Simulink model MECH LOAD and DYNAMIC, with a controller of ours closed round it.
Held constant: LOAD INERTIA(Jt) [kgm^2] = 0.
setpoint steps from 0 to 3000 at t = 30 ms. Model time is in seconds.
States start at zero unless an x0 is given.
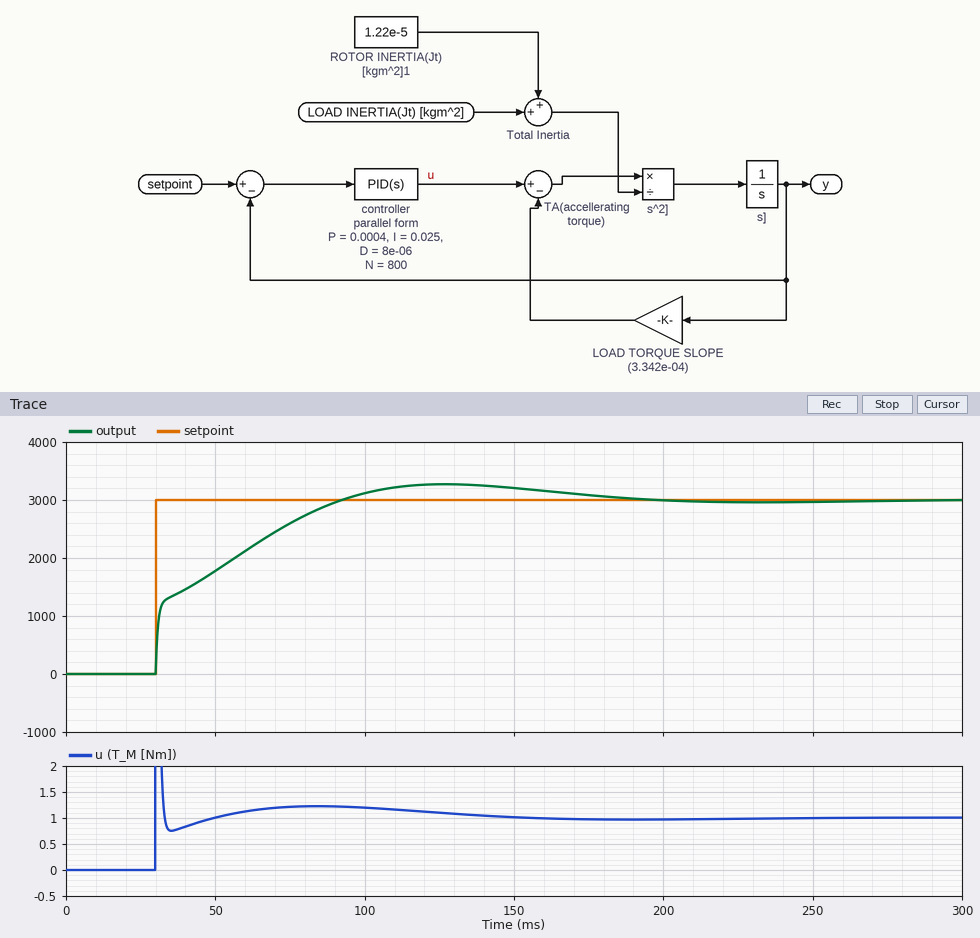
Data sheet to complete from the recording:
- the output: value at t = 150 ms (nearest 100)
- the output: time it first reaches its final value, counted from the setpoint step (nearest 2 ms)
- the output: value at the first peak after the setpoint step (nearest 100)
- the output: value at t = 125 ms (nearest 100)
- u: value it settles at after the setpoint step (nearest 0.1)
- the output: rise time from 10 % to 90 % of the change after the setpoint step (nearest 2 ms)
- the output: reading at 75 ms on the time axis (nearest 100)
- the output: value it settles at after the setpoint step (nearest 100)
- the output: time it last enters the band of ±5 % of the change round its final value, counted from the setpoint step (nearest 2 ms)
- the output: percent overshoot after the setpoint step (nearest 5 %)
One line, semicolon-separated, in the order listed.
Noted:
3200; 62 ms; 3300; 3300; 1.0; 48 ms; 2600; 3000; 132 ms; 10 %
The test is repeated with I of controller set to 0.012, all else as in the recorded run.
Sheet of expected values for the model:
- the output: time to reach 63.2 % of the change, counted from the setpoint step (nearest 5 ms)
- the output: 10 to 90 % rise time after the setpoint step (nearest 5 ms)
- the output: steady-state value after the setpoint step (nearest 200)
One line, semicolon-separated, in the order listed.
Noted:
35 ms; 85 ms; 3000
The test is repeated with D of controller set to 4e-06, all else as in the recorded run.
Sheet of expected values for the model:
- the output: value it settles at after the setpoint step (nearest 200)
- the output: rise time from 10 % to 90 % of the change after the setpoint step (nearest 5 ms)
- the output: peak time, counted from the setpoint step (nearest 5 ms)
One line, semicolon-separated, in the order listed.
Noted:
3000; 40 ms; 85 ms
